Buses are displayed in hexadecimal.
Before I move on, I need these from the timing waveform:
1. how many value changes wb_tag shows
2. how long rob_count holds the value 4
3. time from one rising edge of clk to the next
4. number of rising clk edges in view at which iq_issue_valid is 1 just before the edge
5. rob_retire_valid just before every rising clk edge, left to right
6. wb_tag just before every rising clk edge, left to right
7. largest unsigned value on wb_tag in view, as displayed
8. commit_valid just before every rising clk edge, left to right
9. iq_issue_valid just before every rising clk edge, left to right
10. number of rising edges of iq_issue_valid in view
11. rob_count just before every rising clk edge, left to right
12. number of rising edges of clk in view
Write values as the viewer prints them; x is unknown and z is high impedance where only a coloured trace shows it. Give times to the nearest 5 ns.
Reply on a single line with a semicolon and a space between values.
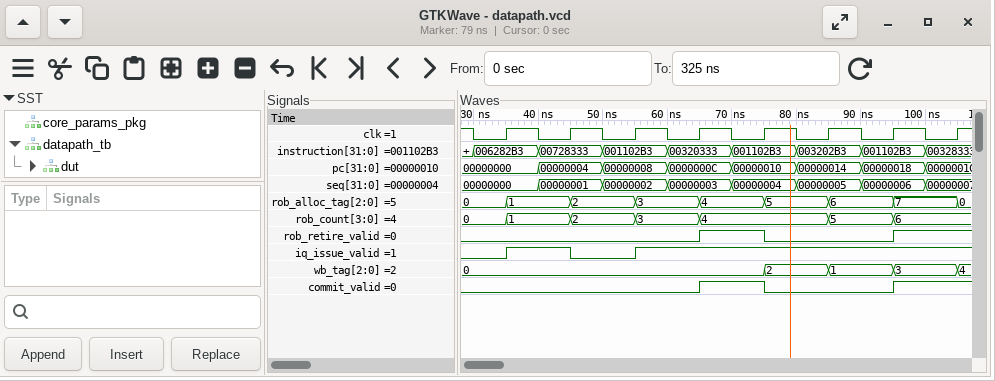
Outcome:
4; 20 ns; 10 ns; 6; 0 0 0 0 1 0 0 1; 0, 0, 0, 0, 0, 2, 1, 3; 4; 0 0 0 0 1 0 0 1; 0 1 0 1 1 1 1 1; 2; 0, 1, 2, 3, 4, 4, 5, 6; 8
